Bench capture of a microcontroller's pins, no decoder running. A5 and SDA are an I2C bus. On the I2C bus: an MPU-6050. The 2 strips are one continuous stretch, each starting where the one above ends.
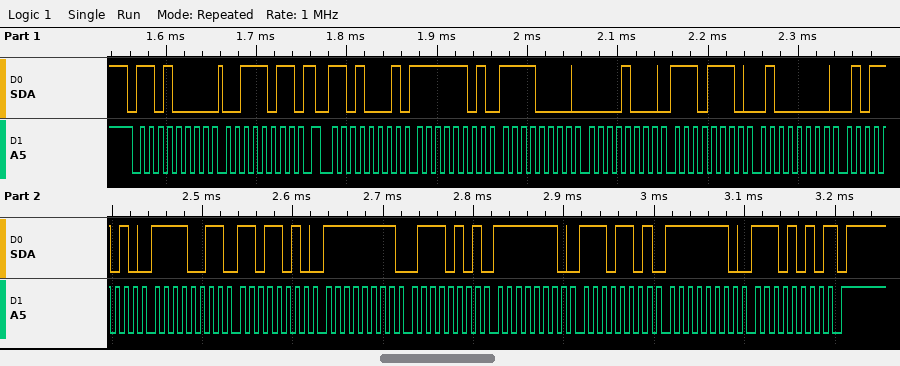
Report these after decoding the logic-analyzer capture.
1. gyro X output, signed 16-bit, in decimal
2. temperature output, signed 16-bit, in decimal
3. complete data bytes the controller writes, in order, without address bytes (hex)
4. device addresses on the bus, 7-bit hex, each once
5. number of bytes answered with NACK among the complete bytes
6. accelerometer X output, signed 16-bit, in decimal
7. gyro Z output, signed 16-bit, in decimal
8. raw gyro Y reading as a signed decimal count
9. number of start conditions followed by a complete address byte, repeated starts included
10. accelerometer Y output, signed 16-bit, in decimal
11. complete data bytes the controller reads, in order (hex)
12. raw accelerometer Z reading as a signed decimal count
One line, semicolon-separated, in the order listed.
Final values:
-139; -3110; 3B; 0x68; 1; -528; -278; -275; 2; 2286; FD F0 08 EE 40 5A F3 DA FF 75 FE ED FE EA; 16474
